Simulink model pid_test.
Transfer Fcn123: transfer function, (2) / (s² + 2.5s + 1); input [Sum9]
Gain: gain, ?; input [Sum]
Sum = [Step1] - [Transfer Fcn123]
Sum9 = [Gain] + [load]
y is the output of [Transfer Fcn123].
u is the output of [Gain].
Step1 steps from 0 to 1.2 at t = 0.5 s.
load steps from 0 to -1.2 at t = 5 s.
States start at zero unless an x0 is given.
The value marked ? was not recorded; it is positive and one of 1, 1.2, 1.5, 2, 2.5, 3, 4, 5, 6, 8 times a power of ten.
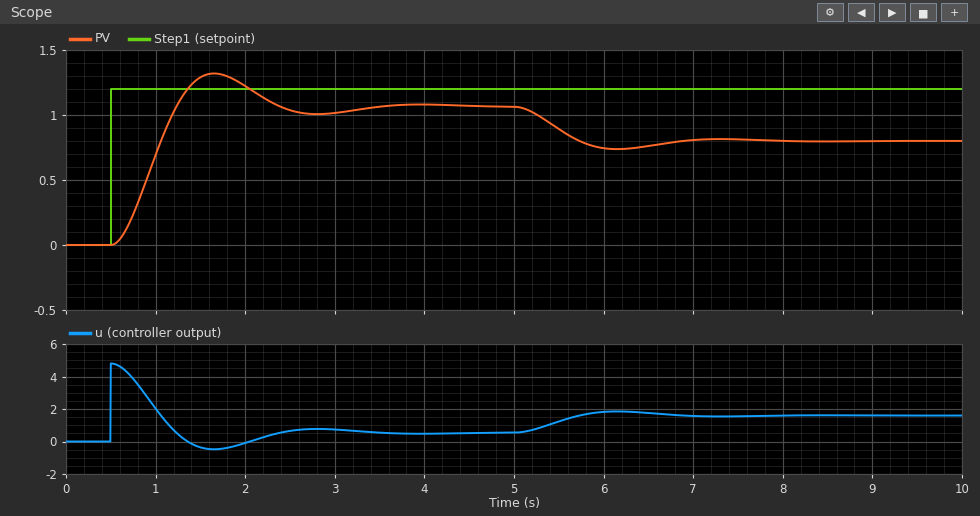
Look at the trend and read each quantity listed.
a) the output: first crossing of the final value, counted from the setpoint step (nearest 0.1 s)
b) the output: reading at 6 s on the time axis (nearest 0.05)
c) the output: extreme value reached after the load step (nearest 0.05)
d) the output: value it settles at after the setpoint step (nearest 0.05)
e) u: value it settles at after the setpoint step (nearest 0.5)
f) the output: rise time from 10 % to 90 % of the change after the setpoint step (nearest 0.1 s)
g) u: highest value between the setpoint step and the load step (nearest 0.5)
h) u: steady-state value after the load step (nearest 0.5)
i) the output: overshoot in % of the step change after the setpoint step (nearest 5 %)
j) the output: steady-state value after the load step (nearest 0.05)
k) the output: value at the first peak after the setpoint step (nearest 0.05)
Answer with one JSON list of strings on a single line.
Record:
["0.7 s", "0.75", "0.75", "1.05", "0.5", "0.5 s", "5.0", "1.5", "25 %", "0.80", "1.30"]
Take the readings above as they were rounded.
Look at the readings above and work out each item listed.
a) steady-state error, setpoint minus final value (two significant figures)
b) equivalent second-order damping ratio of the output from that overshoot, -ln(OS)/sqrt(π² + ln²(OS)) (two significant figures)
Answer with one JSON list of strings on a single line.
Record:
["0.15", "0.40"]
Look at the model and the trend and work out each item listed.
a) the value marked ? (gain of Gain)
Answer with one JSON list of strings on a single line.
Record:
["4"]
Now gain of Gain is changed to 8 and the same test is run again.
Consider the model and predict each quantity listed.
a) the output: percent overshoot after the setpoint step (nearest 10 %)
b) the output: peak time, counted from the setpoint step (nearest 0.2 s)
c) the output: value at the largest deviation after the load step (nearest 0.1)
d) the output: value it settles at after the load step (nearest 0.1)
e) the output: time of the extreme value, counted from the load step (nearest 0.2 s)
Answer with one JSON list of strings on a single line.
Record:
["40 %", "0.8 s", "0.9", "1.0", "0.8 s"]
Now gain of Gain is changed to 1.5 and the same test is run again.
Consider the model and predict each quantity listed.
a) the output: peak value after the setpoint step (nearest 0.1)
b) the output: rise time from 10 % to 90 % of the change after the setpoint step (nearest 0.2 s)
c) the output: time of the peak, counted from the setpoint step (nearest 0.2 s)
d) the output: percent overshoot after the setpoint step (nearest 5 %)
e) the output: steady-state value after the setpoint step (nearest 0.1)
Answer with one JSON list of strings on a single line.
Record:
["1.0", "1.0 s", "2.0 s", "10 %", "0.9"]
